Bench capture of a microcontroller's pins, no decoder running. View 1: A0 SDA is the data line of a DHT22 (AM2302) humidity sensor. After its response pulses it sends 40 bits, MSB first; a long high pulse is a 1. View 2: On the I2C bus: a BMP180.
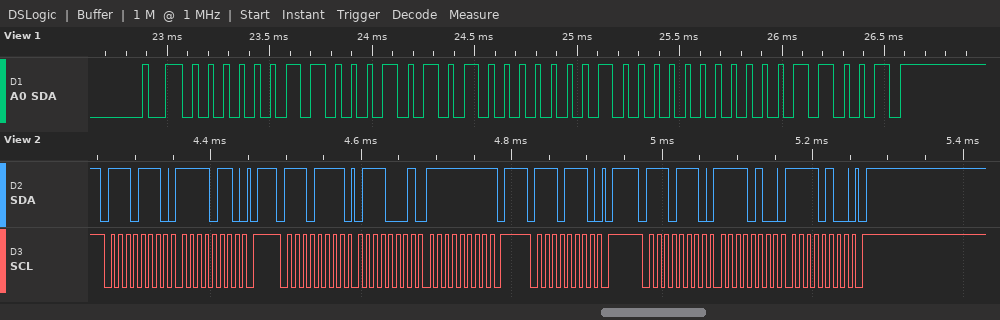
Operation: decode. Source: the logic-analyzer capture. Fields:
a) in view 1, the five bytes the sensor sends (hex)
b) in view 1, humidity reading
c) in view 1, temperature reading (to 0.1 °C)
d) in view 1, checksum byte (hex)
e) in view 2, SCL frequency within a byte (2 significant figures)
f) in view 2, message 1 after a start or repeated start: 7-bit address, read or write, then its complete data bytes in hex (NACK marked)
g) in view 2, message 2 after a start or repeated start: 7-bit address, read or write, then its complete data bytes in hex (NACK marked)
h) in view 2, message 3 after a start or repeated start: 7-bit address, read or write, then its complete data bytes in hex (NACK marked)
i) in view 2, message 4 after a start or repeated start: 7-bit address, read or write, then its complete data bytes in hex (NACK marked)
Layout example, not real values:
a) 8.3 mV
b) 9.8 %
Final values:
a) 03 15 01 00 19
b) 78.9 %
c) 25.6 °C
d) 0x19
e) 100 kHz
f) 0x77 write: F6
g) 0x77 read: 71 FF NACK
h) 0x77 write
i) 0x77 write: F4 F4
